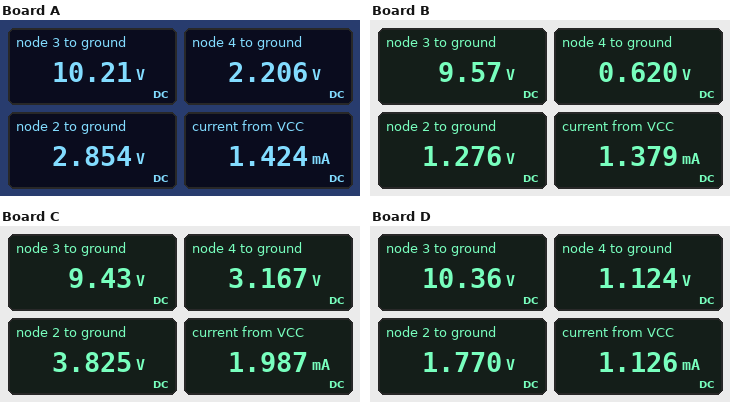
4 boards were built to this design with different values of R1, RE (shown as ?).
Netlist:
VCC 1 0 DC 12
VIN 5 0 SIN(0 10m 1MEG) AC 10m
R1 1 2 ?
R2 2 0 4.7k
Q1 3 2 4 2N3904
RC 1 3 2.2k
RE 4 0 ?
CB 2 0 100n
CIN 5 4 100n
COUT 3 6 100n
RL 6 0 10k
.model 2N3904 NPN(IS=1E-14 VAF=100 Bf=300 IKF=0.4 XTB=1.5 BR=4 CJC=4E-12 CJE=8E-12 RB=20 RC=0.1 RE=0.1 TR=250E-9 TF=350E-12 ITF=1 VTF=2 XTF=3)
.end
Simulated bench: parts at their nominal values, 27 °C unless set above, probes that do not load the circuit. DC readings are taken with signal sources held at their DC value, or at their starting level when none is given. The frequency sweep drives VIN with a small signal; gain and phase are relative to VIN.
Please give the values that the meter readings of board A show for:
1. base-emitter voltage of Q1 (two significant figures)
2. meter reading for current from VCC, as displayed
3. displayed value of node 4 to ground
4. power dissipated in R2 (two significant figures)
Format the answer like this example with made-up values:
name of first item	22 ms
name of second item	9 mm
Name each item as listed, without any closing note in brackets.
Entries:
base-emitter voltage of Q1	650 mV
meter reading for current from VCC, as displayed	1.424 mA
displayed value of node 4 to ground	2.206 V
power dissipated in R2	1.7 mW
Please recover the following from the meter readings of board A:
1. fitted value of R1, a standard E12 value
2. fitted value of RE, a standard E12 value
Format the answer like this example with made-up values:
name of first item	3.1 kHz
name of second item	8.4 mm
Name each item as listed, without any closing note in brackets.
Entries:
fitted value of R1, a standard E12 value	15 kΩ
fitted value of RE, a standard E12 value	2.7 kΩ
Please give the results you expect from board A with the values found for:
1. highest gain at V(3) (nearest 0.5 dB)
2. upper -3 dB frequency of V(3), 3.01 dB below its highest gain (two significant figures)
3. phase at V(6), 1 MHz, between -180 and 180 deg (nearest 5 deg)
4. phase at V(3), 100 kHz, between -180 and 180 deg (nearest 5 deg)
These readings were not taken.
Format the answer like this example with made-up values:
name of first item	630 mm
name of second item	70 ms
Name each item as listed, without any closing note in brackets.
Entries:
highest gain at V(3)	35.0 dB
upper -3 dB frequency of V(3), 3.01 dB below its highest gain	29 MHz
phase at V(6), 1 MHz, between -180 and 180 deg	0 deg
phase at V(3), 100 kHz, between -180 and 180 deg	25 deg
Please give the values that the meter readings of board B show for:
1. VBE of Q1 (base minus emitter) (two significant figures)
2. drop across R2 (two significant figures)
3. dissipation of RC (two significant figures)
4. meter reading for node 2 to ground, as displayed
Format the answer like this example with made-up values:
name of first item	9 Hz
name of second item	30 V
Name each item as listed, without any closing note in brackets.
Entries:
VBE of Q1 (base minus emitter)	660 mV
drop across R2	1.3 V
dissipation of RC	2.7 mW
meter reading for node 2 to ground, as displayed	1.276 V
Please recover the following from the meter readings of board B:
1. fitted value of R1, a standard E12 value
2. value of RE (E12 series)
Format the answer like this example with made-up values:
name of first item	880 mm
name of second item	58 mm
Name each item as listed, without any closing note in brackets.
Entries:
fitted value of R1, a standard E12 value	39 kΩ
value of RE	560 Ω
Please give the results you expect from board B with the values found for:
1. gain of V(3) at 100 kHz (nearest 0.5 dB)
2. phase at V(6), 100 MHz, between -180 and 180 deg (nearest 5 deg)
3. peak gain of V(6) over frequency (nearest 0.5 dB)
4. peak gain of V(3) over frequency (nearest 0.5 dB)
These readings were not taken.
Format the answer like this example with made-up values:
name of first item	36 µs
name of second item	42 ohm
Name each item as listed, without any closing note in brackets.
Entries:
gain of V(3) at 100 kHz	36.0 dB
phase at V(6), 100 MHz, between -180 and 180 deg	-85 deg
peak gain of V(6) over frequency	37.5 dB
peak gain of V(3) over frequency	37.5 dB
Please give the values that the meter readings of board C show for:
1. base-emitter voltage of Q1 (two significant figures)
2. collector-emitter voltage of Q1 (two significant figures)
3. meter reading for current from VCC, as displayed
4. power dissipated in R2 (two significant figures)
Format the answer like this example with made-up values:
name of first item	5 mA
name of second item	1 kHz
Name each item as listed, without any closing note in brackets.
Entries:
base-emitter voltage of Q1	660 mV
collector-emitter voltage of Q1	6.3 V
meter reading for current from VCC, as displayed	1.987 mA
power dissipated in R2	3.1 mW
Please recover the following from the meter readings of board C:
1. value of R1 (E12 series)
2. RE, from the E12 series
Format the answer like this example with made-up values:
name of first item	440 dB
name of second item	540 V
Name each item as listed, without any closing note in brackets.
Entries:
value of R1	10 kΩ
RE, from the E12 series	2.7 kΩ
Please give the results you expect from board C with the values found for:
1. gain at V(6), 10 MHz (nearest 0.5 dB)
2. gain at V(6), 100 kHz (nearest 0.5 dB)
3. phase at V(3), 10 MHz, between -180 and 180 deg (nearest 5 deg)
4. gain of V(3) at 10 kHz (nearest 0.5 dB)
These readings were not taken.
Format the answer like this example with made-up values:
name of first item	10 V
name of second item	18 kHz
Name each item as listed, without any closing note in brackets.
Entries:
gain at V(6), 10 MHz	37.0 dB
gain at V(6), 100 kHz	36.0 dB
phase at V(3), 10 MHz, between -180 and 180 deg	-25 deg
gain of V(3) at 10 kHz	21.0 dB
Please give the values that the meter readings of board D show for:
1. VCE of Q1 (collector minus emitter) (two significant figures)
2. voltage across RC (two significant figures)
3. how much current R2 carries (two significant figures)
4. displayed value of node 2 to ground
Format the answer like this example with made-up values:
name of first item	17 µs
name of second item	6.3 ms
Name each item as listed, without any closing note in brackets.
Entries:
VCE of Q1 (collector minus emitter)	9.2 V
voltage across RC	1.6 V
how much current R2 carries	380 µA
displayed value of node 2 to ground	1.770 V
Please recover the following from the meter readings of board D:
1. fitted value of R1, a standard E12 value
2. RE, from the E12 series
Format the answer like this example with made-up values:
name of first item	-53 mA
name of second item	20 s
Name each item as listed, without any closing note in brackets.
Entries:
fitted value of R1, a standard E12 value	27 kΩ
RE, from the E12 series	1.5 kΩ
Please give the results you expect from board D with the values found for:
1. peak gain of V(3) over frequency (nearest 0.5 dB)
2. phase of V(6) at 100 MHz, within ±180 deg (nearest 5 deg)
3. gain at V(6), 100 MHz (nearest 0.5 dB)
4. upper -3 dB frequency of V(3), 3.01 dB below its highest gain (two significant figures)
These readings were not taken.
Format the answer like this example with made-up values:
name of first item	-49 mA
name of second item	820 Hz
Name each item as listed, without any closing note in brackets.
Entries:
peak gain of V(3) over frequency	34.0 dB
phase of V(6) at 100 MHz, within ±180 deg	-80 deg
gain at V(6), 100 MHz	23.5 dB
upper -3 dB frequency of V(3), 3.01 dB below its highest gain	31 MHz
